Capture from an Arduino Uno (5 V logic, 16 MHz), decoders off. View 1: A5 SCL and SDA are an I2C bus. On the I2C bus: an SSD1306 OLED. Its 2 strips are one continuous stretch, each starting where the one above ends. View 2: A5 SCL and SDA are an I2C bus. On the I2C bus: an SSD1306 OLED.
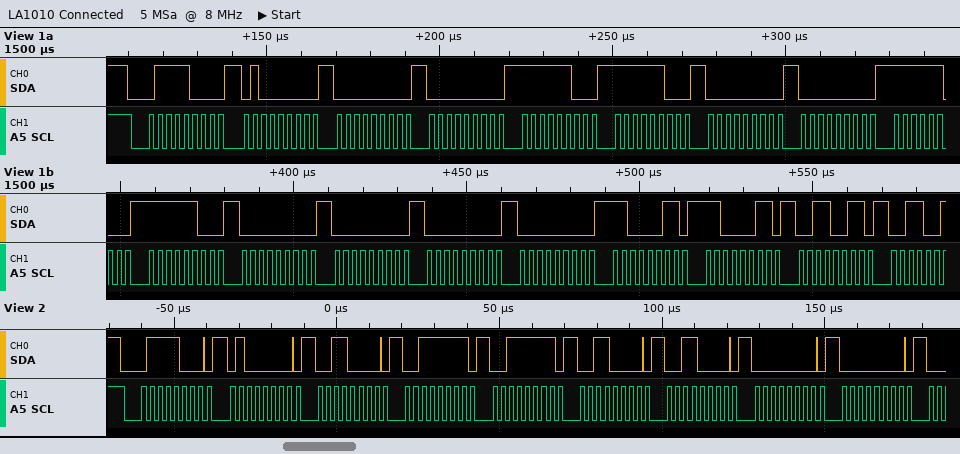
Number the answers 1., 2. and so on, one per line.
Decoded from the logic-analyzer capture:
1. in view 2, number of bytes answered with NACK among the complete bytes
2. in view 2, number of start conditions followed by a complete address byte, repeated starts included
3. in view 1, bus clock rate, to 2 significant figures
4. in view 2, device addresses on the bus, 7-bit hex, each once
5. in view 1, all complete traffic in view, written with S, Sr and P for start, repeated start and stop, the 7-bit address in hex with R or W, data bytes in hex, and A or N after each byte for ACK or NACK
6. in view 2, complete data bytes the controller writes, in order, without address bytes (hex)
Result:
1. 0
2. 1
3. 400 kHz
4. 0x3C
5. S 3CW A 40 A 00 A 00 A FC A FC A 00 A 00 A FC A FC A 00 A 00 A 00 A 00 A C3 A C3 A 33 A
6. 40 30 3F 3F 30 30 00 00
